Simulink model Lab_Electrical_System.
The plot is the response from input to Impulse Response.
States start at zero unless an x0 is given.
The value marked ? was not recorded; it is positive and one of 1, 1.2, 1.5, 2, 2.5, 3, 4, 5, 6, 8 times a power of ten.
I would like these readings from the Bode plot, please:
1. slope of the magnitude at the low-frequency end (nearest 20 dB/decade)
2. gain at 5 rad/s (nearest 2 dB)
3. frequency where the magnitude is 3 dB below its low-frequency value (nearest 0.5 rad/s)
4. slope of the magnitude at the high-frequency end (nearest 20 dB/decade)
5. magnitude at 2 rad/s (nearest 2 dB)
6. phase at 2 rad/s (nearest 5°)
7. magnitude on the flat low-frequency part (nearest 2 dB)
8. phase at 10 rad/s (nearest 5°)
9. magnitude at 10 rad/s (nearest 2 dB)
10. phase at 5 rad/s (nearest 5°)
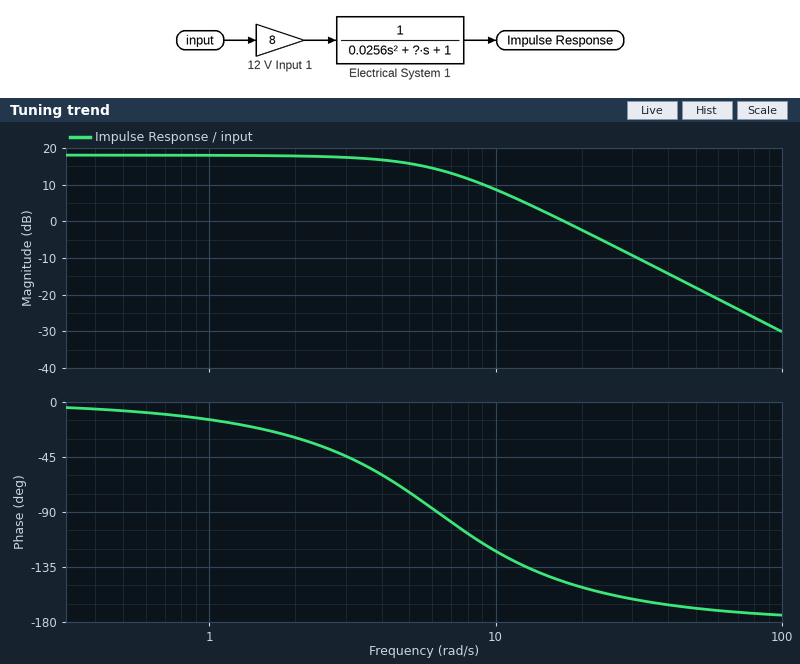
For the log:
0 dB/decade
16 dB
5.5 rad/s
-40 dB/decade
18 dB
-30°
18 dB
-120°
8 dB
-75°
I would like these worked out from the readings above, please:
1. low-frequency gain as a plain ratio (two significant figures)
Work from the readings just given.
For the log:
7.9
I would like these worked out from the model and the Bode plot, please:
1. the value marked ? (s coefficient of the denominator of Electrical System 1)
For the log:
0.25
